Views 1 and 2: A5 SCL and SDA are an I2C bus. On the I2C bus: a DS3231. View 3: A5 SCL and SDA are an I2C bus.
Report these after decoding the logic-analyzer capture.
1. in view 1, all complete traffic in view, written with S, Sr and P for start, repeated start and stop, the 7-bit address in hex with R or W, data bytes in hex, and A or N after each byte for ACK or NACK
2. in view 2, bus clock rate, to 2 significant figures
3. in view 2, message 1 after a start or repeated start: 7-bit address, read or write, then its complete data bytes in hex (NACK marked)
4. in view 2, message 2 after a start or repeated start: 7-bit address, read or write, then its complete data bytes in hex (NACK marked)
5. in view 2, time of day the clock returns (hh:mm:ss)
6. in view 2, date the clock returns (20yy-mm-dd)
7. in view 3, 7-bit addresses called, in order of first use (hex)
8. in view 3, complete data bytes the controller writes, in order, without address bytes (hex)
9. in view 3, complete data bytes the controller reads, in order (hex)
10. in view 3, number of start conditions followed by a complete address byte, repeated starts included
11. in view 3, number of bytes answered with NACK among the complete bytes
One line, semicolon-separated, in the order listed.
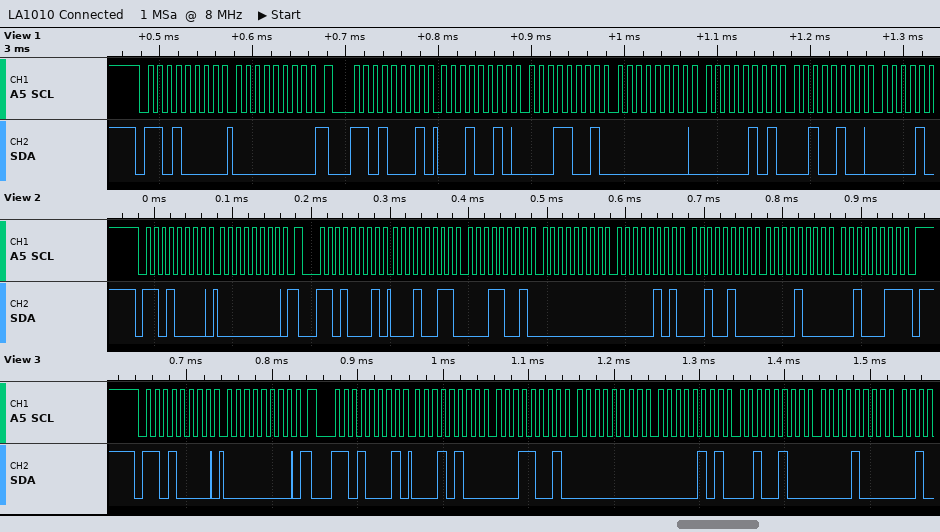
S 68W A 00 A Sr 68R A 12 A 19 A 00 A 05 A 24 A; 100 kHz; 0x68 write: 00; 0x68 read: 13 19 00 05 24 08 23 NACK; 00:19:13; 2023-08-24; 0x68; 00; 14 19 00 05 24 08; 2; 0
